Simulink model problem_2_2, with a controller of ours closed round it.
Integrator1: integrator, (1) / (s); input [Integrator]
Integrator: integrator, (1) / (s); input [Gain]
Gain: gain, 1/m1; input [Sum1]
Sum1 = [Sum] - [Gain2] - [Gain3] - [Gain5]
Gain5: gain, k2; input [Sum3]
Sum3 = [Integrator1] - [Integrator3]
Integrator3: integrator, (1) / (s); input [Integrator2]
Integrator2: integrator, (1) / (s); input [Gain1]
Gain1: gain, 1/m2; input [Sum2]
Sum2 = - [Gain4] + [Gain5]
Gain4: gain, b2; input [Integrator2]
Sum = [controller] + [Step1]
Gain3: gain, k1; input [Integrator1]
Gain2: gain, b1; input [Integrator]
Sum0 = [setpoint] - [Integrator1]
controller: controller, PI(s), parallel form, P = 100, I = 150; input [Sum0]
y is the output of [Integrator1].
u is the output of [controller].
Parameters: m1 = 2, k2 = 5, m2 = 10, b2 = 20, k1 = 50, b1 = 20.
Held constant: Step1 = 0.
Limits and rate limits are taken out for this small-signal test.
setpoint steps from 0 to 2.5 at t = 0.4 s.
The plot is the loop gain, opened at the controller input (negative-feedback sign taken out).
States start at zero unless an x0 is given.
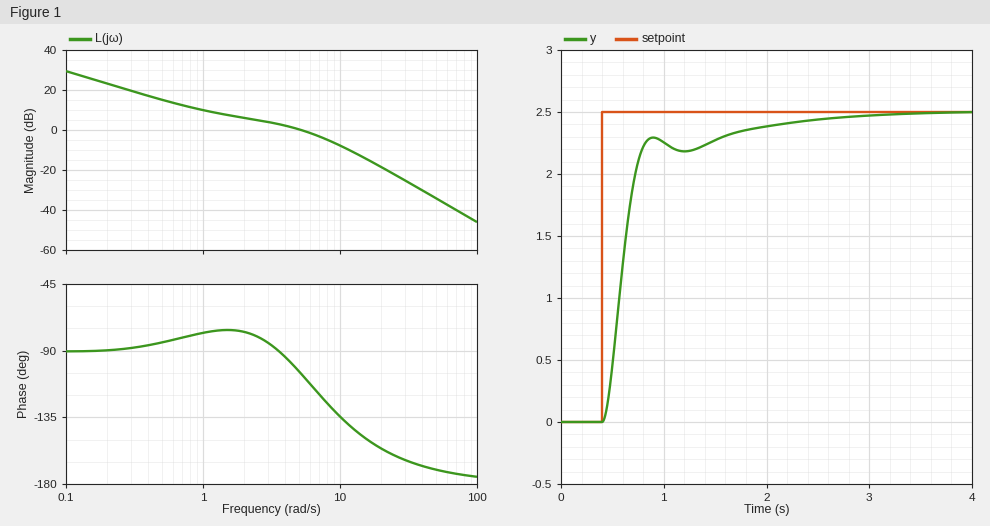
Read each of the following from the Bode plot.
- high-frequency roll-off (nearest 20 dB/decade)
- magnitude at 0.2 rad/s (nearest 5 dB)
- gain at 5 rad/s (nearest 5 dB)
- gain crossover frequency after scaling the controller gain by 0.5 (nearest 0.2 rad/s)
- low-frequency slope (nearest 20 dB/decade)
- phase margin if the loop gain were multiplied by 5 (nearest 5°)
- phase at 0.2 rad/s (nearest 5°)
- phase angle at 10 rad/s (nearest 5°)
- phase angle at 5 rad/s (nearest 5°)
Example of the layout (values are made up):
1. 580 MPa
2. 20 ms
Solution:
1. -40 dB/decade
2. 25 dB
3. 0 dB
4. 2.0 rad/s
5. -20 dB/decade
6. 30°
7. -90°
8. -135°
9. -105°
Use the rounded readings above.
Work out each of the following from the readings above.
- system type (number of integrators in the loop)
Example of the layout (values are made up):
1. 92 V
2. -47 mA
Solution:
1. 1
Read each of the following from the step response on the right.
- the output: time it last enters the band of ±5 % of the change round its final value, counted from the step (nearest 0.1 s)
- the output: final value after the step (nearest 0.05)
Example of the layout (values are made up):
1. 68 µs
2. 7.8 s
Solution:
1. 1.5 s
2. 2.50
